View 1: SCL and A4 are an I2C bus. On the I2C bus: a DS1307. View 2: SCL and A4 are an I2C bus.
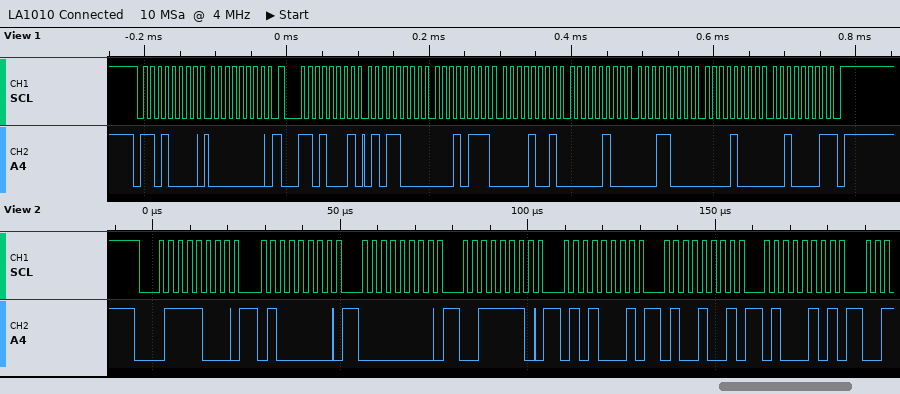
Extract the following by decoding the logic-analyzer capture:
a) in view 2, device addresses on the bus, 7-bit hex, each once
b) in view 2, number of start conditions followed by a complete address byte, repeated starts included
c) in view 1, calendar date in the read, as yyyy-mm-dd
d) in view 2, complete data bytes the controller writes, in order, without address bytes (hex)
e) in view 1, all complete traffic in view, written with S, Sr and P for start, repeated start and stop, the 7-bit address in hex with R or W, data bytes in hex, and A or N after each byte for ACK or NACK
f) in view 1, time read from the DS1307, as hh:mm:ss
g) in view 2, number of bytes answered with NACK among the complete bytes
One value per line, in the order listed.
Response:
0x3C
1
2021-08-18
40 00 3E 51 49 45
S 68W A 00 A Sr 68R A 58 A 17 A 09 A 04 A 18 A 08 A 21 N P
09:17:58
0
